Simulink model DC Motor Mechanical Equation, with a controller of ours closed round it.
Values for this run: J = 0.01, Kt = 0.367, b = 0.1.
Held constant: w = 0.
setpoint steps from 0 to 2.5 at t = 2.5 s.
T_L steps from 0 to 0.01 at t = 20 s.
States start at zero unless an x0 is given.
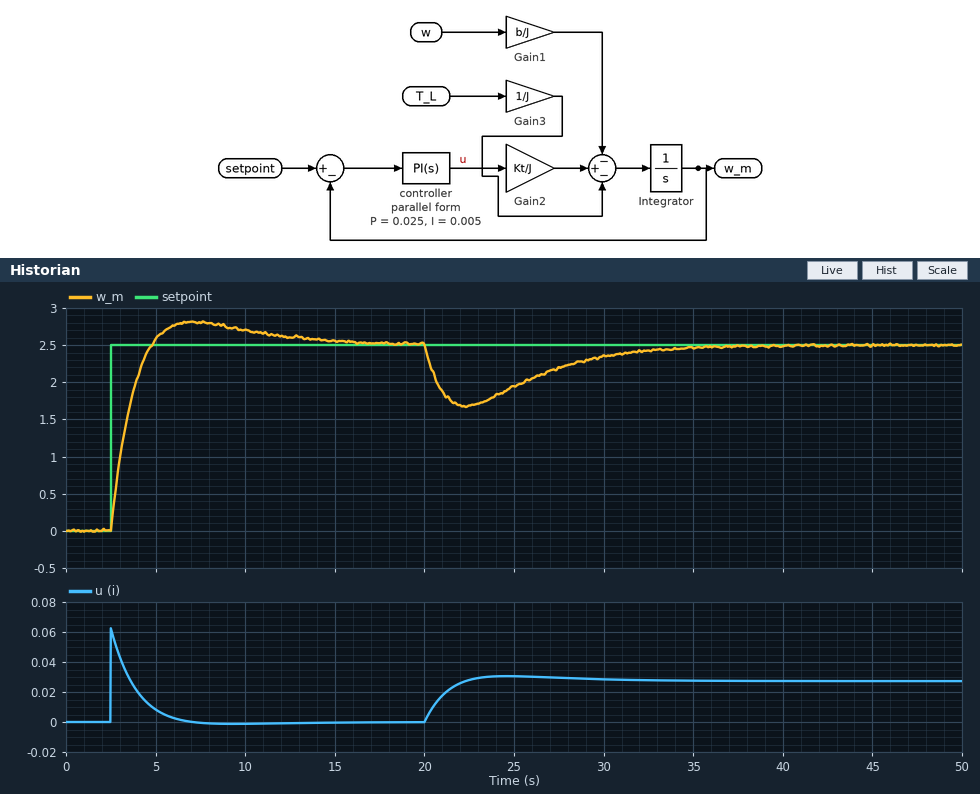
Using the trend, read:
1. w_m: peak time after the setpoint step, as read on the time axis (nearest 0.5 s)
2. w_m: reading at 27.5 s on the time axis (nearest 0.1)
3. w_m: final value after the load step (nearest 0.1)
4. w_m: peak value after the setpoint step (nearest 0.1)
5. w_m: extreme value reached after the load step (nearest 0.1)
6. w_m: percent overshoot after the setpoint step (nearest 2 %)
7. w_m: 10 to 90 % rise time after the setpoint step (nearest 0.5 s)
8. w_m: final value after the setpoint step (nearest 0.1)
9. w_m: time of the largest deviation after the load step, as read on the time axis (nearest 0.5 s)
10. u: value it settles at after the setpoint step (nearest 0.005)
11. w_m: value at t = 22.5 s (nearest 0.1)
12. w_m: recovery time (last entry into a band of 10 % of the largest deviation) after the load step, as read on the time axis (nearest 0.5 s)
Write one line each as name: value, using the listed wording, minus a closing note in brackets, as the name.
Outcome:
w_m: peak time after the setpoint step, as read on the time axis: 7.0 s
w_m: reading at 27.5 s on the time axis: 2.2
w_m: final value after the load step: 2.5
w_m: peak value after the setpoint step: 2.8
w_m: extreme value reached after the load step: 1.7
w_m: percent overshoot after the setpoint step: 12 %
w_m: 10 to 90 % rise time after the setpoint step: 1.5 s
w_m: final value after the setpoint step: 2.5
w_m: time of the largest deviation after the load step, as read on the time axis: 22.5 s
u: value it settles at after the setpoint step: 0.000
w_m: value at t = 22.5 s: 1.7
w_m: recovery time (last entry into a band of 10 % of the largest deviation) after the load step, as read on the time axis: 32.0 s
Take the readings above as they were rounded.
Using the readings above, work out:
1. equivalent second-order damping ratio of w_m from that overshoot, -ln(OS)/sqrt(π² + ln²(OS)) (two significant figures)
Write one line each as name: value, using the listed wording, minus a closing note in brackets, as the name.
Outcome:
equivalent second-order damping ratio of w_m from that overshoot, -ln(OS)/sqrt(π² + ln²(OS)): 0.56
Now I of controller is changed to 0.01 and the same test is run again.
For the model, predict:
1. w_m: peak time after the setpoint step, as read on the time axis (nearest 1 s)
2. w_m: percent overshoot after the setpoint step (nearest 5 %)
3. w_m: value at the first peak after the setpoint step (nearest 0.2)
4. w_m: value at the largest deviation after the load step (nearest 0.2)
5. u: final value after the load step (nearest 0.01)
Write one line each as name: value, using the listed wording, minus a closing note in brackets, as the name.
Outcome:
w_m: peak time after the setpoint step, as read on the time axis: 6 s
w_m: percent overshoot after the setpoint step: 20 %
w_m: value at the first peak after the setpoint step: 3.0
w_m: value at the largest deviation after the load step: 1.8
u: final value after the load step: 0.03
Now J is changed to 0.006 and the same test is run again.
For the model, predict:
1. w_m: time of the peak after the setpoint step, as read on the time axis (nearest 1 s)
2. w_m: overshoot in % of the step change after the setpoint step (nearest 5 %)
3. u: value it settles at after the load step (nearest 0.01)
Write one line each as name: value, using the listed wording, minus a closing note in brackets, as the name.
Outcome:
w_m: time of the peak after the setpoint step, as read on the time axis: 6 s
w_m: overshoot in % of the step change after the setpoint step: 10 %
u: value it settles at after the load step: 0.03
